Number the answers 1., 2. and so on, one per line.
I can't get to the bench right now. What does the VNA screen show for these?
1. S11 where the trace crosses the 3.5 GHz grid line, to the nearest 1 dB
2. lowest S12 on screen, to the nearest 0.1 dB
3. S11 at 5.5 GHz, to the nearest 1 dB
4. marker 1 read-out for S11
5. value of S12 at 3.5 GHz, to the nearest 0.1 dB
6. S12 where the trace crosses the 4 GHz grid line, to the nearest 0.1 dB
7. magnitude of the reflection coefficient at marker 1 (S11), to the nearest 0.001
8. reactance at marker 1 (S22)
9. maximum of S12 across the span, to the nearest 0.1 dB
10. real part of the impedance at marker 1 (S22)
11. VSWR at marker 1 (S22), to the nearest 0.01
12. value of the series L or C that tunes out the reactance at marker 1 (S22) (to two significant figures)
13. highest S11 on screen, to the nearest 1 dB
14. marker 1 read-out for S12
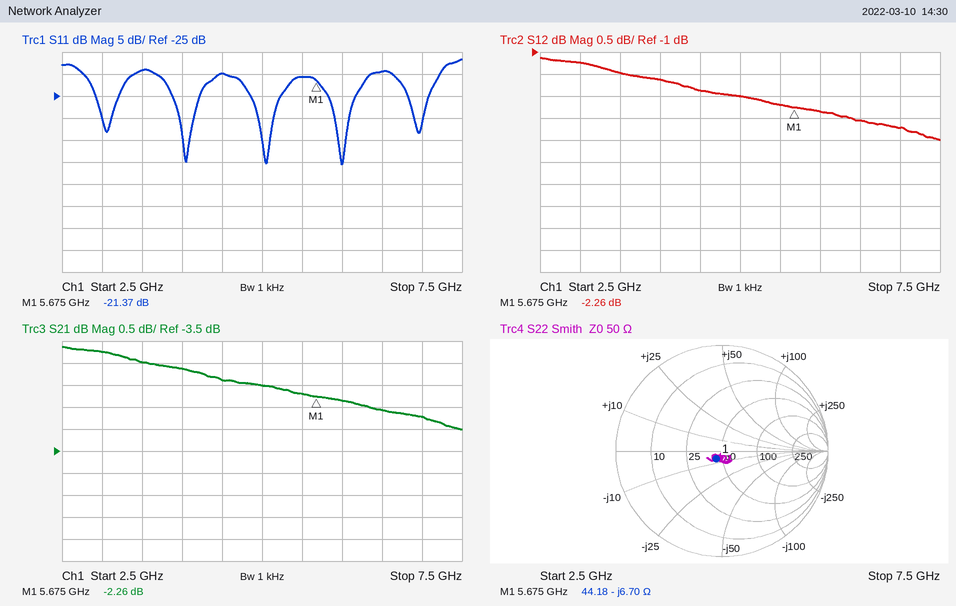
1. -19 dB
2. -3.0 dB
3. -21 dB
4. -21.37 dB
5. -1.5 dB
6. -1.6 dB
7. 0.085
8. -6.70 Ω
9. -1.1 dB
10. 44.18 Ω
11. 1.21
12. 190 pH
13. -17 dB
14. -2.26 dB
